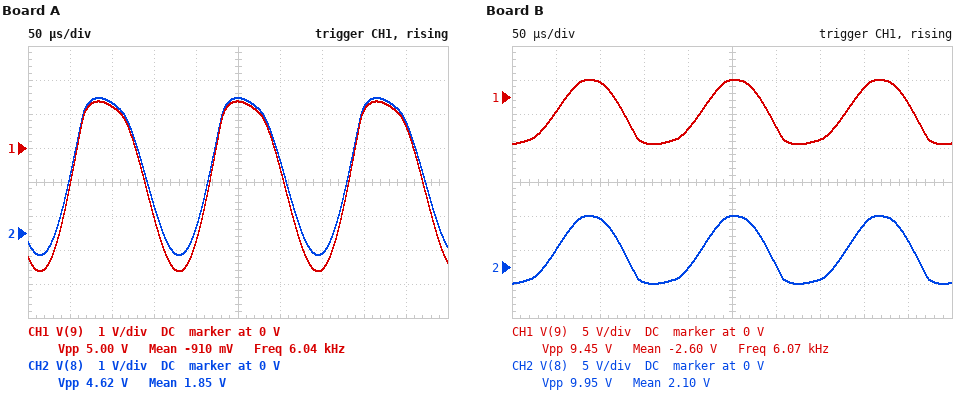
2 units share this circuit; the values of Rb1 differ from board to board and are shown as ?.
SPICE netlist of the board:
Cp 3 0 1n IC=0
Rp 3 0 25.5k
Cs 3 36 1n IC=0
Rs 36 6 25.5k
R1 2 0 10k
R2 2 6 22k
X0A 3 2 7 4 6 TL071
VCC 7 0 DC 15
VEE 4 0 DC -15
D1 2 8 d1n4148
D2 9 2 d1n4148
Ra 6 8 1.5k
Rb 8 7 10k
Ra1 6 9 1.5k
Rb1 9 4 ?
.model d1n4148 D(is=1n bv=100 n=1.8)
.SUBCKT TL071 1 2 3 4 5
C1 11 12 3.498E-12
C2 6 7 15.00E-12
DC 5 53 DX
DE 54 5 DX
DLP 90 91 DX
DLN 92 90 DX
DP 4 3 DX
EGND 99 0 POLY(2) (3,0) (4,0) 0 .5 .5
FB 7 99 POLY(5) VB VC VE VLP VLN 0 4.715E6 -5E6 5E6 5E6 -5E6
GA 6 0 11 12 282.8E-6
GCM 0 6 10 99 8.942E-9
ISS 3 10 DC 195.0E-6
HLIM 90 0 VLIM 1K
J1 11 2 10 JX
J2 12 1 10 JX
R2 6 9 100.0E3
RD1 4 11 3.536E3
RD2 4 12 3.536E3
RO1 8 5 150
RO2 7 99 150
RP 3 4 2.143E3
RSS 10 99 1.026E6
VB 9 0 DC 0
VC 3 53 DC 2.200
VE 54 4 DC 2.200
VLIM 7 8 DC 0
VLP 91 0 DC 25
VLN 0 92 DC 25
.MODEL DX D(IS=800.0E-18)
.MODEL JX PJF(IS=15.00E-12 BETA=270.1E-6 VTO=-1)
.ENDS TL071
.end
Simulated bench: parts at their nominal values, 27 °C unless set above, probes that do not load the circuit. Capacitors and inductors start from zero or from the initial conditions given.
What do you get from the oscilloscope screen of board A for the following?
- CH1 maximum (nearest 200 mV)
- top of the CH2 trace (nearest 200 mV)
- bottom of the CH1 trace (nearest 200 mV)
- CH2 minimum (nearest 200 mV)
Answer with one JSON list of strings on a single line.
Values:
["1.4 V", "4.0 V", "-3.6 V", "-600 mV"]
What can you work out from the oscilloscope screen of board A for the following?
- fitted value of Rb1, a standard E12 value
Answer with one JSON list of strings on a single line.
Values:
["27 kΩ"]
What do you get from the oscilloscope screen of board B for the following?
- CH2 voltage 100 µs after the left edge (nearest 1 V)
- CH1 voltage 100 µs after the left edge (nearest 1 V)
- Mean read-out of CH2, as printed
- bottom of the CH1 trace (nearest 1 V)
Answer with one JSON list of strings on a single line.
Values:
["7 V", "2 V", "2.10 V", "-7 V"]
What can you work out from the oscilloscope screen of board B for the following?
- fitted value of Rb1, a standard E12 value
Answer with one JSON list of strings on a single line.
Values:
["6.8 kΩ"]
